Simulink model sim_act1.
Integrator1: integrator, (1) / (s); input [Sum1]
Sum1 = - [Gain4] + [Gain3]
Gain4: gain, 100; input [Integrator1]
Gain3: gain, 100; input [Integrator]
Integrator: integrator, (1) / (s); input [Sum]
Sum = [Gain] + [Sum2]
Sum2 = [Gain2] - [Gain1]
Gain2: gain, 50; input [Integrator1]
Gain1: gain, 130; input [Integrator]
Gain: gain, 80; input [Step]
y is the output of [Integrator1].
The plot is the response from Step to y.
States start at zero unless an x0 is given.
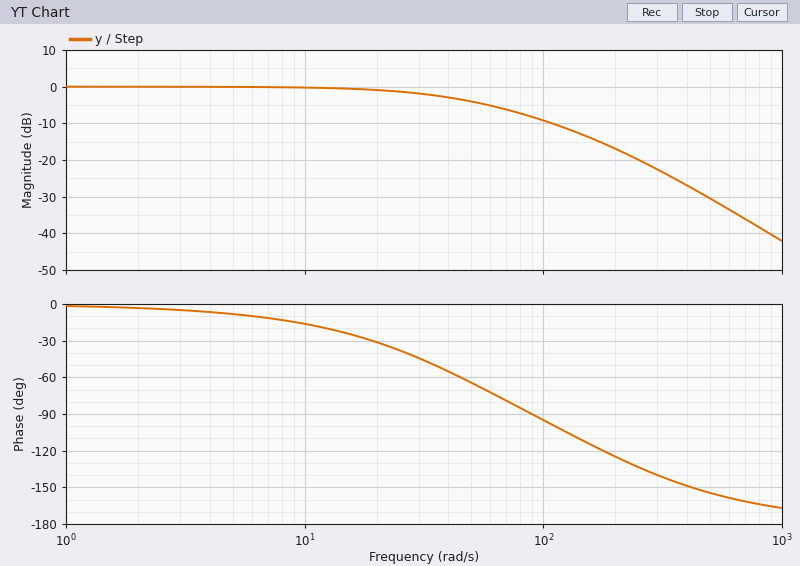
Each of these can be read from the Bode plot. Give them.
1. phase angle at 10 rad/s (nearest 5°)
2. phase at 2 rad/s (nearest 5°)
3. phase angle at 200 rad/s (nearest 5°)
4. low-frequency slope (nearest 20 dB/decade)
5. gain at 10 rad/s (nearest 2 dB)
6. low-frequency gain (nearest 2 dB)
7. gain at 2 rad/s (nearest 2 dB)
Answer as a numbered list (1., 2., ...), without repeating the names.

1. -15°
2. -5°
3. -125°
4. 0 dB/decade
5. 0 dB
6. 0 dB
7. 0 dB
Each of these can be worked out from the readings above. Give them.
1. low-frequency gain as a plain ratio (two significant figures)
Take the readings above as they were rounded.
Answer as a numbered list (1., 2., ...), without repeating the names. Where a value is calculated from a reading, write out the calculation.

1. 10^(0 / 20) = 1.0
